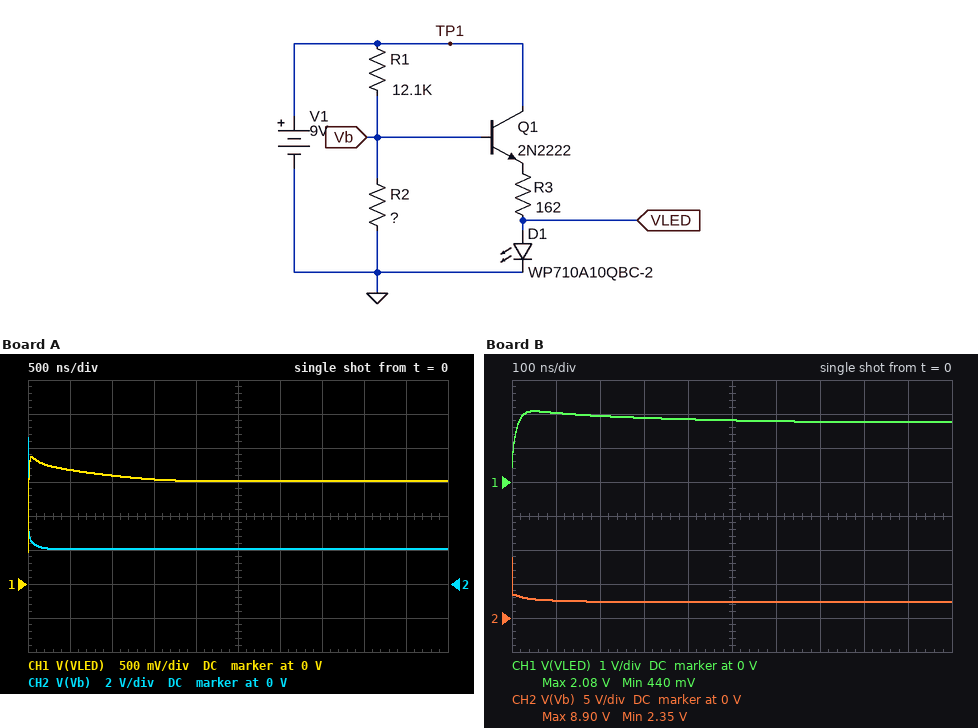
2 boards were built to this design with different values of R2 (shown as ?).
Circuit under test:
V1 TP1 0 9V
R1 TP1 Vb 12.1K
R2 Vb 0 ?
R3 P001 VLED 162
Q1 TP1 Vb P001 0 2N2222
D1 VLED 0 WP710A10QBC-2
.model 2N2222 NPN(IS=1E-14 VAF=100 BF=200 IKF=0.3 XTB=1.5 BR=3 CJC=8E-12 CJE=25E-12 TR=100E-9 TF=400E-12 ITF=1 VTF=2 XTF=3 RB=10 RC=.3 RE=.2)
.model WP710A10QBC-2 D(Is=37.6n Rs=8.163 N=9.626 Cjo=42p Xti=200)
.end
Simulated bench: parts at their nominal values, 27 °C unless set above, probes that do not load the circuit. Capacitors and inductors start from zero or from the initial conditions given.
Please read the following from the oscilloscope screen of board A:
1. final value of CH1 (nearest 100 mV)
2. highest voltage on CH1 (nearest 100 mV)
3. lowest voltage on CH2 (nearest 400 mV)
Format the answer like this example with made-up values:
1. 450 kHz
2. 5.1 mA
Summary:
1. 1.5 V
2. 1.9 V
3. 2.0 V
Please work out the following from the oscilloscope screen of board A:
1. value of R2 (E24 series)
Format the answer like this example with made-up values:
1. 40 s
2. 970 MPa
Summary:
1. 3.6 kΩ
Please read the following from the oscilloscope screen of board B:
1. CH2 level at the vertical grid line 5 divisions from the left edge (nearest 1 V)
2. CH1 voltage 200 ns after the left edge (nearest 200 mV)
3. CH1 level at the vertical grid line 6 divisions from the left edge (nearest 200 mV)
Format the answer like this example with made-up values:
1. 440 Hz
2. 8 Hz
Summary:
1. 2 V
2. 2.0 V
3. 1.8 V
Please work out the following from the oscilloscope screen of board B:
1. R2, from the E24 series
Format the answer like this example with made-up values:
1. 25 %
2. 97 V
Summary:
1. 4.3 kΩ
